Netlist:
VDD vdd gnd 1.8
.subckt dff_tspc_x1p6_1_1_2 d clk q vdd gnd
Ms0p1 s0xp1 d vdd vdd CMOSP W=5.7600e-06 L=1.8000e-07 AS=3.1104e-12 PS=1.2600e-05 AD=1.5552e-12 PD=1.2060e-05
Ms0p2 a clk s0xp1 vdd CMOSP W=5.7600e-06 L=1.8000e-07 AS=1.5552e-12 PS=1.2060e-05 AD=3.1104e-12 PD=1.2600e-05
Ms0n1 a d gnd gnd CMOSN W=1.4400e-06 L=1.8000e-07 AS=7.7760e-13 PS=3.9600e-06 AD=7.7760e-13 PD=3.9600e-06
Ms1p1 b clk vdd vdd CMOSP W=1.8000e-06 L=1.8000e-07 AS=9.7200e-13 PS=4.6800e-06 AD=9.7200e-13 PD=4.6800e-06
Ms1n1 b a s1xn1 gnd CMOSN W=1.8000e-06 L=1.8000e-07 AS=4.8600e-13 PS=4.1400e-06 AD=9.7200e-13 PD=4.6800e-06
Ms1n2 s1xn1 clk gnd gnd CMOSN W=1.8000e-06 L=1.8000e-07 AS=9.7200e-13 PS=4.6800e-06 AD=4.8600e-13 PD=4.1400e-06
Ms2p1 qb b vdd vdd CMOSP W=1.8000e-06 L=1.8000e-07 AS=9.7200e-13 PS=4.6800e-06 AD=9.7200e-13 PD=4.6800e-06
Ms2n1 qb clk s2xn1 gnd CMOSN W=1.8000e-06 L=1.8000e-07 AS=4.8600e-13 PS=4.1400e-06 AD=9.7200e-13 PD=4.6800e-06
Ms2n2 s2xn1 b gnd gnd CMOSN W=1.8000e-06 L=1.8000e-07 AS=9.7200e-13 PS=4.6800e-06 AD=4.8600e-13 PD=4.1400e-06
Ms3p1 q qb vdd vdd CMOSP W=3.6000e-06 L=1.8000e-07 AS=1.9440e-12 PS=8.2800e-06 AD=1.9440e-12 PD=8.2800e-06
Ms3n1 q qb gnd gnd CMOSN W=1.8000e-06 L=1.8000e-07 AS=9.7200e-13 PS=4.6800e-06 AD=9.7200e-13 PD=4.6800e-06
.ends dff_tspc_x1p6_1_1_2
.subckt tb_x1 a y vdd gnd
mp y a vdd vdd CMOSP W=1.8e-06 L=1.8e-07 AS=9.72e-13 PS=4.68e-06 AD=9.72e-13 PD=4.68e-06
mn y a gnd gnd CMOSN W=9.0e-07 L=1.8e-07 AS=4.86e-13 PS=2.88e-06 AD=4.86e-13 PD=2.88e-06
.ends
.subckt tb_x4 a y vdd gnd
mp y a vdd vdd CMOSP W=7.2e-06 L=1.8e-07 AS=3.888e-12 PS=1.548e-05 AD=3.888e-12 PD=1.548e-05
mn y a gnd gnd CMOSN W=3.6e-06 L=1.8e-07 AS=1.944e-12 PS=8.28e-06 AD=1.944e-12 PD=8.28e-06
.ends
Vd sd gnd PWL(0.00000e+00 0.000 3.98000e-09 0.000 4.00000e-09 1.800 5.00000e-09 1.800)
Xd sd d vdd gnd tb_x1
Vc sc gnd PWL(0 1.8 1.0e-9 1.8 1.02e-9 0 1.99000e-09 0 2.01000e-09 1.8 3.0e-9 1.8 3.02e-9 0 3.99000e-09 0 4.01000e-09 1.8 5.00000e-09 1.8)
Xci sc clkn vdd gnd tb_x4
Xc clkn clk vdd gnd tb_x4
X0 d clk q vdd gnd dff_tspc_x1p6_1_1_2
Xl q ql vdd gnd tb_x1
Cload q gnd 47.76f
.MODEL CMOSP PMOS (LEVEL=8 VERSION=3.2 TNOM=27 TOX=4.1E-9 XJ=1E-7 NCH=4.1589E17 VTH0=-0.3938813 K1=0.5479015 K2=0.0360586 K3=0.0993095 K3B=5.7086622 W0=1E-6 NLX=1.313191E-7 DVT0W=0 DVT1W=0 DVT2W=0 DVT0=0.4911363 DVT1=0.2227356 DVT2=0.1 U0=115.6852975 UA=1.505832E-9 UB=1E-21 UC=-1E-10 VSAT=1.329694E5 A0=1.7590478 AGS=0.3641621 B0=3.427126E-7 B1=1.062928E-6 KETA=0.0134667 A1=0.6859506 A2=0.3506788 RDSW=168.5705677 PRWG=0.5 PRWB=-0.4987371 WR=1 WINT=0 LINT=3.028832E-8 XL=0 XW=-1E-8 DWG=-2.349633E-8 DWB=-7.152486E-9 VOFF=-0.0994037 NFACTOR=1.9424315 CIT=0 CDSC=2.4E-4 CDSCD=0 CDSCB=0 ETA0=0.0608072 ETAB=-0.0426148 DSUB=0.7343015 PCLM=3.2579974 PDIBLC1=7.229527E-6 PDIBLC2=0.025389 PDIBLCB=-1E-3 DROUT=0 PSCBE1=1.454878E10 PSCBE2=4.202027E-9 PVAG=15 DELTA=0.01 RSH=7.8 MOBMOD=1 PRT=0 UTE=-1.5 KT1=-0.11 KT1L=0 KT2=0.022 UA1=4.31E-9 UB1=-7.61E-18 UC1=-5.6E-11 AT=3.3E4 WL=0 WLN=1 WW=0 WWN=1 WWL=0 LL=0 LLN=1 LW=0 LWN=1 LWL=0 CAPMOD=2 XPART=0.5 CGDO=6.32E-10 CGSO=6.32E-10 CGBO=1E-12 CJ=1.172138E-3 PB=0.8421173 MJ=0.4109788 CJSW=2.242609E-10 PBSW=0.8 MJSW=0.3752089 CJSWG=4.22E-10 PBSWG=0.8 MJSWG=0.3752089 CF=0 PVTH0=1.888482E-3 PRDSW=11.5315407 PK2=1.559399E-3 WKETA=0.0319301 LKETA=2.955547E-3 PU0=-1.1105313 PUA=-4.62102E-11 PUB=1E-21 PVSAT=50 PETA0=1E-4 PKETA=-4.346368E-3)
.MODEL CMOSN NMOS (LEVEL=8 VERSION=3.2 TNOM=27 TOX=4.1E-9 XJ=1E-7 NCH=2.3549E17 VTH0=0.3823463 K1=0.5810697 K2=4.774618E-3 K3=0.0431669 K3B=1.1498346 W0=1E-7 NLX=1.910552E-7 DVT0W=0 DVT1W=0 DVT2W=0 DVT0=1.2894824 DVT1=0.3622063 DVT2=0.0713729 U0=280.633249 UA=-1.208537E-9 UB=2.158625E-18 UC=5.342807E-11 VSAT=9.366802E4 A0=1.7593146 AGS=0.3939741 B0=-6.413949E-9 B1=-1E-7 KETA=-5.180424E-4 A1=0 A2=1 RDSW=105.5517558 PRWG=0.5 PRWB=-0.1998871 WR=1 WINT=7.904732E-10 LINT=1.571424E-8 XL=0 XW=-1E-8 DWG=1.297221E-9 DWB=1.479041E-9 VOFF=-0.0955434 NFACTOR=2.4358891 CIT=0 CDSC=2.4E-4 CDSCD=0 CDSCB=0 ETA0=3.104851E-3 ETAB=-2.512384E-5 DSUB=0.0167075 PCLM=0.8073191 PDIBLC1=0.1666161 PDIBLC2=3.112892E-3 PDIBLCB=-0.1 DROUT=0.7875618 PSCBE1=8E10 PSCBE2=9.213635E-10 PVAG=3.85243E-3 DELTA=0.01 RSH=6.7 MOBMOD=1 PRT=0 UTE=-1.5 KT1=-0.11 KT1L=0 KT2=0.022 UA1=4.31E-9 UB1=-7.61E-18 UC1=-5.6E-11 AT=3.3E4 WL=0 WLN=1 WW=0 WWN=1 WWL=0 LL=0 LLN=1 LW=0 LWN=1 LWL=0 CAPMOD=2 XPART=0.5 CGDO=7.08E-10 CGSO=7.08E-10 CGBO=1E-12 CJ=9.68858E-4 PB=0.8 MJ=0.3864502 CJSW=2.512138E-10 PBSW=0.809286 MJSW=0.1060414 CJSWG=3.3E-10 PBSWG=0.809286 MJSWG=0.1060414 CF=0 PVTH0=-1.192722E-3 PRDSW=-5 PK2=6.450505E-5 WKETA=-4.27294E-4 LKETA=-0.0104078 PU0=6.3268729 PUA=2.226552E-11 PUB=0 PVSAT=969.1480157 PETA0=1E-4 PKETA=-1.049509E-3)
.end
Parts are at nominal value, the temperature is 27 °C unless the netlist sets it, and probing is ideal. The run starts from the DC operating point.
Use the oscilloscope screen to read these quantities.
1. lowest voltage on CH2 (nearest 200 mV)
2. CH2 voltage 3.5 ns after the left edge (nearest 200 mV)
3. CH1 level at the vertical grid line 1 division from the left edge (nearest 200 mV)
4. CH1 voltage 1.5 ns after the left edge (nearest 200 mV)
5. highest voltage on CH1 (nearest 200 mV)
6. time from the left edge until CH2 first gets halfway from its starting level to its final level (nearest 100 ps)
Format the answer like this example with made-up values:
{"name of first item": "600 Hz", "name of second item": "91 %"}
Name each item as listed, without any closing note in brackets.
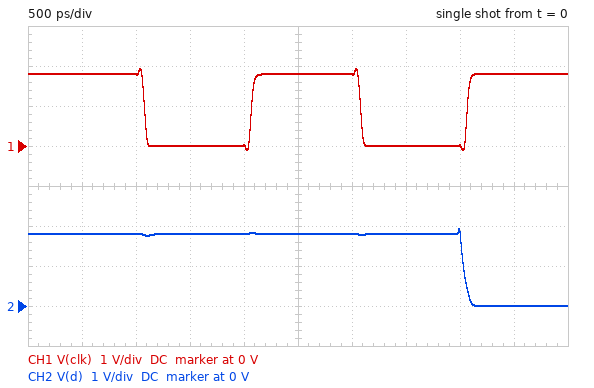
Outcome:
{"lowest voltage on CH2": "0 V", "CH2 voltage 3.5 ns after the left edge": "1.8 V", "CH1 level at the vertical grid line 1 division from the left edge": "1.8 V", "CH1 voltage 1.5 ns after the left edge": "0 V", "highest voltage on CH1": "2.0 V", "time from the left edge until CH2 first gets halfway from its starting level to its final level": "4.0 ns"}
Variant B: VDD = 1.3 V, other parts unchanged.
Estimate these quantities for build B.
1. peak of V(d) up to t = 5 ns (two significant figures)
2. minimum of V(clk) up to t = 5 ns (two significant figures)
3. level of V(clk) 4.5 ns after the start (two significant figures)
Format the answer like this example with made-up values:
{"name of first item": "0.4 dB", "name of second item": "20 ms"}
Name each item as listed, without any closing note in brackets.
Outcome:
{"peak of V(d) up to t = 5 ns": "1.4 V", "minimum of V(clk) up to t = 5 ns": "-170 mV", "level of V(clk) 4.5 ns after the start": "1.3 V"}
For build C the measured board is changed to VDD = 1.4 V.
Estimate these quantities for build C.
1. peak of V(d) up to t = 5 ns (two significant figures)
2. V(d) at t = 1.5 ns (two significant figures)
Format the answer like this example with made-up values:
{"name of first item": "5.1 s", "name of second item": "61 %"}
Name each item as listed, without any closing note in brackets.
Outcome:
{"peak of V(d) up to t = 5 ns": "1.5 V", "V(d) at t = 1.5 ns": "1.4 V"}
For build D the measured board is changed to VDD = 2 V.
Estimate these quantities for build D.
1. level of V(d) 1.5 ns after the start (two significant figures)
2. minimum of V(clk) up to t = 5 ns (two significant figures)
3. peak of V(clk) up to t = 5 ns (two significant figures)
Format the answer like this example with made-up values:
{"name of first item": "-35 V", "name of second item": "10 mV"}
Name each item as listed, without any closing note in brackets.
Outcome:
{"level of V(d) 1.5 ns after the start": "2.0 V", "minimum of V(clk) up to t = 5 ns": "-100 mV", "peak of V(clk) up to t = 5 ns": "2.1 V"}
